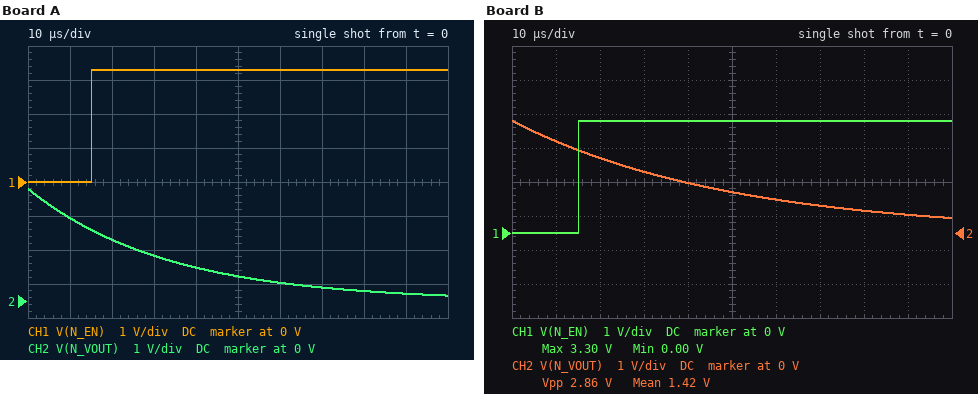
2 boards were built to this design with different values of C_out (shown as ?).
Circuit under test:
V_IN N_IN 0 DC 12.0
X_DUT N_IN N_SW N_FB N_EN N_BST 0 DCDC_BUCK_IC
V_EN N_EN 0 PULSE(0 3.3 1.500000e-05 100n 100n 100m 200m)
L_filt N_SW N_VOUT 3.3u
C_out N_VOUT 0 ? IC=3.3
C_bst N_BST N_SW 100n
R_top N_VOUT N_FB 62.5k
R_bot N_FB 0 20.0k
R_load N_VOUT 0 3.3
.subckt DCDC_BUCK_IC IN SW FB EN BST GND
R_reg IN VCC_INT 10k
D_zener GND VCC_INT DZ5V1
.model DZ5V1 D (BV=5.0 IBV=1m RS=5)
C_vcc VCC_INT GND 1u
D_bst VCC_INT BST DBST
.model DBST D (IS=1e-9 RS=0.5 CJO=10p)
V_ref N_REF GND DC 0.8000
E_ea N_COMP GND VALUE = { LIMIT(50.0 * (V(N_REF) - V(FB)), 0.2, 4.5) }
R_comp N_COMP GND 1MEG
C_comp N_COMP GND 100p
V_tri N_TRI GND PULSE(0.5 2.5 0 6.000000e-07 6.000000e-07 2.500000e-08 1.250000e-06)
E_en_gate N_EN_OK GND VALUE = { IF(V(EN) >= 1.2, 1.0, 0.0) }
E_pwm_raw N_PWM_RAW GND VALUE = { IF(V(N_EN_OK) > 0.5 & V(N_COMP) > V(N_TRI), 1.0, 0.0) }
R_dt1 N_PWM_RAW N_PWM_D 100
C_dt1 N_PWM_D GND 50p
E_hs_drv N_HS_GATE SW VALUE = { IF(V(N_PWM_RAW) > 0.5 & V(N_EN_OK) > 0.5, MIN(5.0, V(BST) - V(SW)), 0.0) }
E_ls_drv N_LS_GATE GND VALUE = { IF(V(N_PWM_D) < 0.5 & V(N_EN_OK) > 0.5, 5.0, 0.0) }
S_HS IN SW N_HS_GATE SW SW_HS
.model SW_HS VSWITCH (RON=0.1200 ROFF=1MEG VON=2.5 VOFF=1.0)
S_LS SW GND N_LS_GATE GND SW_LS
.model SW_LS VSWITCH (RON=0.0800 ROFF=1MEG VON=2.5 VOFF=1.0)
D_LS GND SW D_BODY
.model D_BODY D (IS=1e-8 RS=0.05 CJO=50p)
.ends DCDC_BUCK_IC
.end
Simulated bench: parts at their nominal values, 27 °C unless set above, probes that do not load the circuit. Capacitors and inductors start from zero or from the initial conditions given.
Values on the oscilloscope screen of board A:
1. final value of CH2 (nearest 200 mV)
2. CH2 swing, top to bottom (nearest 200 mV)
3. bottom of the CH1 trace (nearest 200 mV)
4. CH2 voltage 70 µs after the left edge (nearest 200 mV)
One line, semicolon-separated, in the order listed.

200 mV; 3.2 V; 0 V; 400 mV
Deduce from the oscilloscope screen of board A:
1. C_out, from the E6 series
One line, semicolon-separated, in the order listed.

10 µF
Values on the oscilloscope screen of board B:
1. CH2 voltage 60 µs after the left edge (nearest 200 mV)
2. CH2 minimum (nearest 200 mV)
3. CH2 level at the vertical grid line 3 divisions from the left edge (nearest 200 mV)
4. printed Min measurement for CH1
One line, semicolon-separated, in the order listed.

1.0 V; 400 mV; 1.8 V; 0.00 V
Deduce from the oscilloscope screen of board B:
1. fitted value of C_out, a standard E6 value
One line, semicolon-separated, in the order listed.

15 µF
